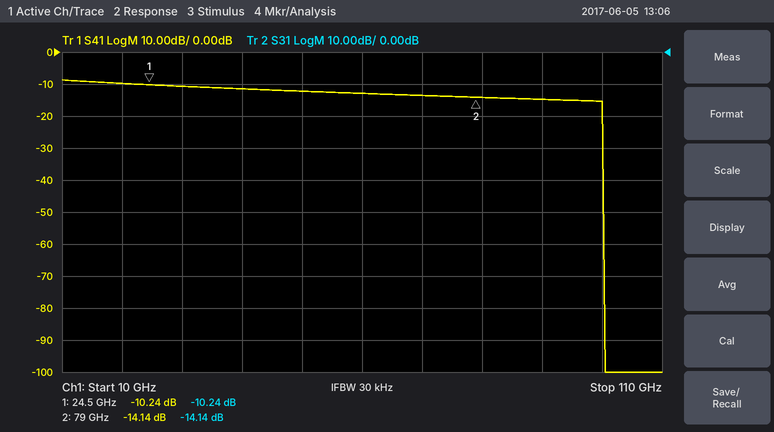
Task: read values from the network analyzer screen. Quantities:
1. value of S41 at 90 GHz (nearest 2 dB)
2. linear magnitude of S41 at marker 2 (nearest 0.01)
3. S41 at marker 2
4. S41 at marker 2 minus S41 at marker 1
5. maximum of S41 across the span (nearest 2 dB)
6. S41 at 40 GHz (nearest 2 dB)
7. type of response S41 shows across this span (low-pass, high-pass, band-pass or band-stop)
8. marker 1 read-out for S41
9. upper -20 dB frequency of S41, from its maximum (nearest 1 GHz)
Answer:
-14 dB
0.20
-14.14 dB
-3.90 dB
-8 dB
-12 dB
low-pass
-10.24 dB
100 GHz
